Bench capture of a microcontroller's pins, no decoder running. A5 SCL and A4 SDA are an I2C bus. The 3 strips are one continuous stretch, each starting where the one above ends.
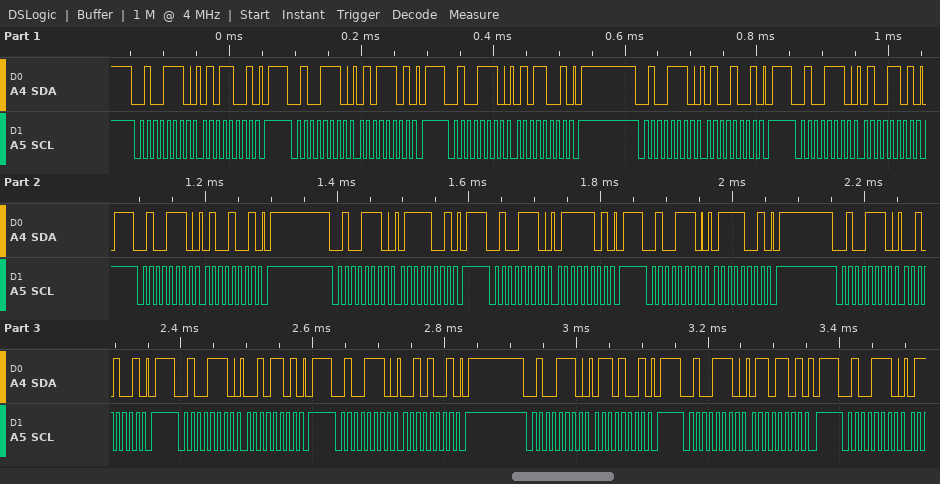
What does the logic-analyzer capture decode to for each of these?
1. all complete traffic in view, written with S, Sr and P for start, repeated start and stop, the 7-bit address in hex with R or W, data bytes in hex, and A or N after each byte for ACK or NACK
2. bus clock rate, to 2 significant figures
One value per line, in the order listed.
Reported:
S 27W A 59 A P S 27W A 5D A P S 27W A 59 A P S 27W A 49 A P S 27W A 4D A P S 27W A 49 A P S 27W A 79 A P S 27W A 7D A P S 27W A 79 A P S 27W A 29 A P S 27W A 2D A P S 27W A 29 A P S 27W A 69 A P S 27W A 6D A P S 27W A
100 kHz
